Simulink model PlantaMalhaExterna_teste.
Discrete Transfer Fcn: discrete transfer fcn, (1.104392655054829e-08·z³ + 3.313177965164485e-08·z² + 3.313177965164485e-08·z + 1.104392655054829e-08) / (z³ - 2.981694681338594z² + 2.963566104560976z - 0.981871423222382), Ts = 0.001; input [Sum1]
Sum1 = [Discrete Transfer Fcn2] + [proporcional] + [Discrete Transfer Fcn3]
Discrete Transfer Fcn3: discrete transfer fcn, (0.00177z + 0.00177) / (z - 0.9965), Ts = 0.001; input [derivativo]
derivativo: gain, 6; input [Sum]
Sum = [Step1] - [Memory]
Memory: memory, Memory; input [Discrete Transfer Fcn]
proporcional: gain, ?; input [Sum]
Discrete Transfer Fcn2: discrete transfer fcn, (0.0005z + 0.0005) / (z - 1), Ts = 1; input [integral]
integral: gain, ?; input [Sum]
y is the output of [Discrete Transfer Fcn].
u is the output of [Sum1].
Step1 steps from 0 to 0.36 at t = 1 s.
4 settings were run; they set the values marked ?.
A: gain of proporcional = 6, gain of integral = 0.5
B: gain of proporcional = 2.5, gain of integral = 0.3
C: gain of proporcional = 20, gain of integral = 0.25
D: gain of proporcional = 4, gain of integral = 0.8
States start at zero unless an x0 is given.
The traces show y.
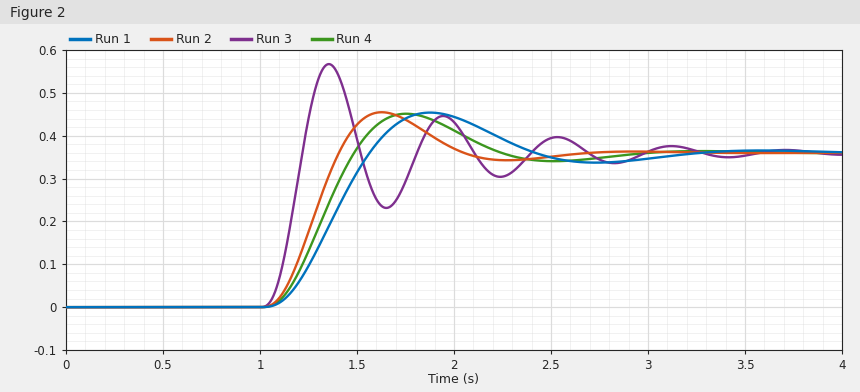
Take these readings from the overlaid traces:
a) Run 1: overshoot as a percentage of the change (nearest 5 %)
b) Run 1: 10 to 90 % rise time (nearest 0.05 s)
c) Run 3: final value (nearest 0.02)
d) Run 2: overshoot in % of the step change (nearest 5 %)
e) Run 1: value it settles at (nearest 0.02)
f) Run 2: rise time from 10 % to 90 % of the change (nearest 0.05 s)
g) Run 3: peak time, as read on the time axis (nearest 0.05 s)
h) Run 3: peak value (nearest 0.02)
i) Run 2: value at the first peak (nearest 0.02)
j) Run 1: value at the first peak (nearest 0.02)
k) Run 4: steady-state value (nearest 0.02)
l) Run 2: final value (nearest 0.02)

25 %
0.35 s
0.36
25 %
0.36
0.25 s
1.35 s
0.56
0.46
0.46
0.36
0.36
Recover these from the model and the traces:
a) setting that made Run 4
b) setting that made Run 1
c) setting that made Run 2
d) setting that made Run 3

D
B
A
C
